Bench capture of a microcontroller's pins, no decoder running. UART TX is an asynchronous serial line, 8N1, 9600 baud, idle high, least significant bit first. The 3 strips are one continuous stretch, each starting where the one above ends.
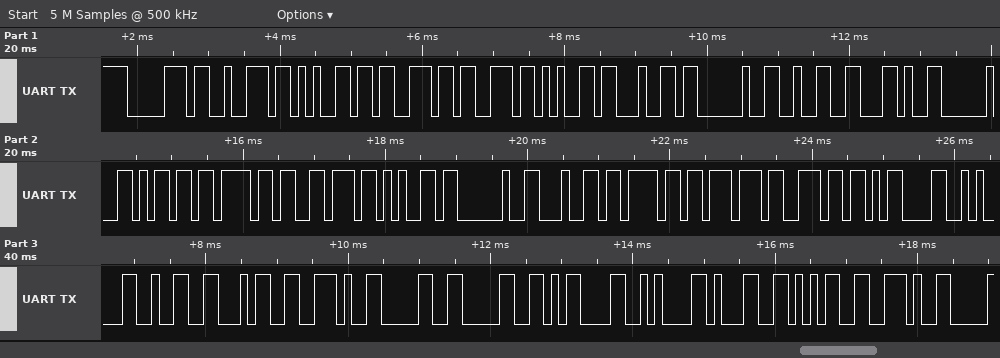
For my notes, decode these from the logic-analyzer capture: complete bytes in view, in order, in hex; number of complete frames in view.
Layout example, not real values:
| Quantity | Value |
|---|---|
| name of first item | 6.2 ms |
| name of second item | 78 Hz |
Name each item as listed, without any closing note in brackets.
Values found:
| Quantity | Value |
|---|---|
| complete bytes in view, in order, in hex | 0x70 0x72 0x65 0x73 0x73 0x65 0x64 0x20 0x32 0x2C 0x20 0x6D 0x6F 0x76 0x65 0x20 0x64 0x6F 0x77 0x6E 0x0D 0x0A 0x32 0x34 0x2E 0x30 0x30 0x0D 0x0A 0x31 0x35 0x2E |
| number of complete frames in view | 32 |
